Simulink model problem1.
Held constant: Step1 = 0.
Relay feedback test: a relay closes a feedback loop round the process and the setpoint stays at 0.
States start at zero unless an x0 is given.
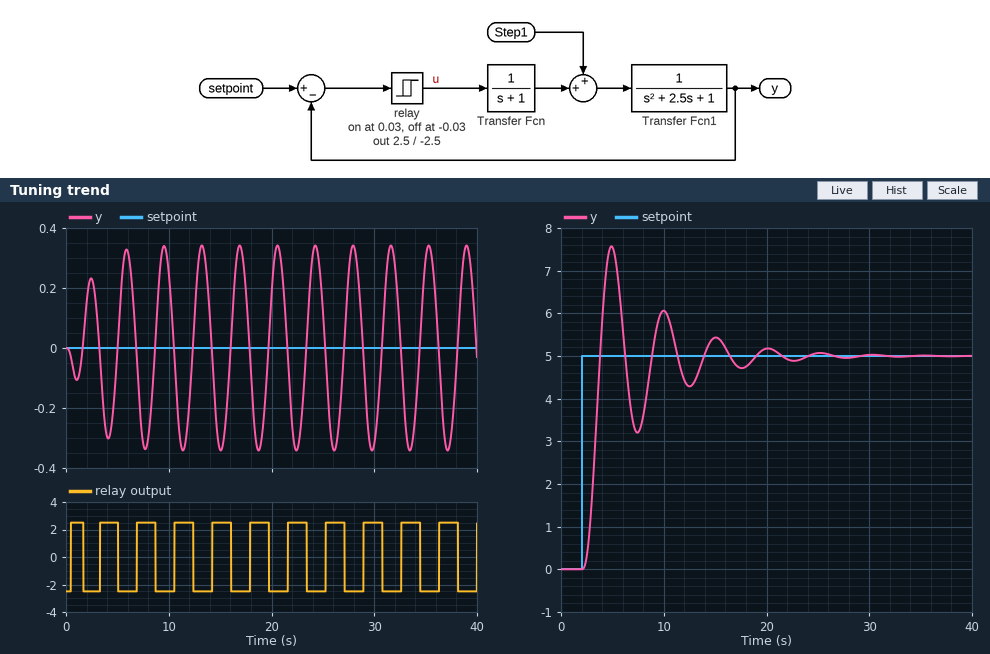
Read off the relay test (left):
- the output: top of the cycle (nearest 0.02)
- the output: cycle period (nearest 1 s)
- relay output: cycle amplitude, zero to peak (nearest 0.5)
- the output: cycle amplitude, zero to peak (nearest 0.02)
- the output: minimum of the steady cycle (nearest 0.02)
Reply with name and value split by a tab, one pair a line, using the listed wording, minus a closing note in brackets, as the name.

the output: top of the cycle	0.34
the output: cycle period	4 s
relay output: cycle amplitude, zero to peak	2.5
the output: cycle amplitude, zero to peak	0.34
the output: minimum of the steady cycle	-0.34
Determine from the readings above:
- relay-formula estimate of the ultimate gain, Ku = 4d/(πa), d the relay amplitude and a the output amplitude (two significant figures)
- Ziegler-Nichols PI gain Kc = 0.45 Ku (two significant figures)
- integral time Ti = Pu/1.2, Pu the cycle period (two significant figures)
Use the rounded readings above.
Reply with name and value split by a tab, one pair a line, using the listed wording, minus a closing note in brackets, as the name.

relay-formula estimate of the ultimate gain, Ku = 4d/(πa), d the relay amplitude and a the output amplitude	9.4
Ziegler-Nichols PI gain Kc = 0.45 Ku	4.2
integral time Ti = Pu/1.2, Pu the cycle period	3.3 s
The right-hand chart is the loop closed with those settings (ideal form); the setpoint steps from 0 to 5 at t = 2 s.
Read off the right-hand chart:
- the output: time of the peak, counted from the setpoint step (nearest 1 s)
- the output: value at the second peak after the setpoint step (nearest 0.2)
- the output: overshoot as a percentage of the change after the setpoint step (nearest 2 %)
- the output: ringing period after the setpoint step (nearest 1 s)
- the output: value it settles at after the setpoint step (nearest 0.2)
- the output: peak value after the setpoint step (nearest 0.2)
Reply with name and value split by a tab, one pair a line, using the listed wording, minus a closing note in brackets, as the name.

the output: time of the peak, counted from the setpoint step	3 s
the output: value at the second peak after the setpoint step	6.0
the output: overshoot as a percentage of the change after the setpoint step	52 %
the output: ringing period after the setpoint step	5 s
the output: value it settles at after the setpoint step	5.0
the output: peak value after the setpoint step	7.6
